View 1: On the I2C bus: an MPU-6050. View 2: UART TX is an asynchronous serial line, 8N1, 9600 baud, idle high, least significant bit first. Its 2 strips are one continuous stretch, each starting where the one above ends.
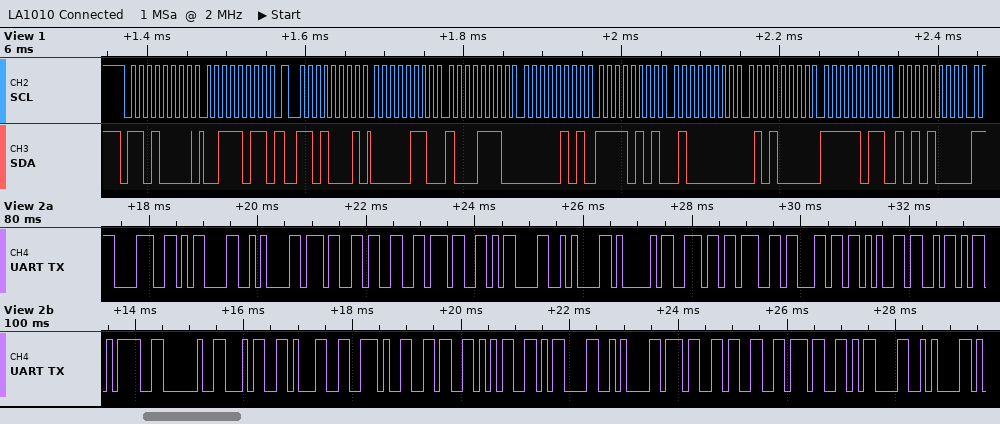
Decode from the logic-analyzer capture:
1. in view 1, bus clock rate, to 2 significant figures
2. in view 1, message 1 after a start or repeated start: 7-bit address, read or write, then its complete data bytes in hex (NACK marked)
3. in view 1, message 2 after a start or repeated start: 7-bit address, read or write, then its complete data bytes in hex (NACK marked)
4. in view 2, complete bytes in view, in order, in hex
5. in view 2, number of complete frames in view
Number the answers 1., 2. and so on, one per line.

1. 100 kHz
2. 0x68 write: 3B
3. 0x68 read: 06 8E 05 F5 40 50 FB A8
4. 38 0D 0A 37 33 37 0D 0A 41 6E 67 6C 65 5A 3D 20 34 31 2E 36 35 0D 0A 37 33 37 0D 0A
5. 28
